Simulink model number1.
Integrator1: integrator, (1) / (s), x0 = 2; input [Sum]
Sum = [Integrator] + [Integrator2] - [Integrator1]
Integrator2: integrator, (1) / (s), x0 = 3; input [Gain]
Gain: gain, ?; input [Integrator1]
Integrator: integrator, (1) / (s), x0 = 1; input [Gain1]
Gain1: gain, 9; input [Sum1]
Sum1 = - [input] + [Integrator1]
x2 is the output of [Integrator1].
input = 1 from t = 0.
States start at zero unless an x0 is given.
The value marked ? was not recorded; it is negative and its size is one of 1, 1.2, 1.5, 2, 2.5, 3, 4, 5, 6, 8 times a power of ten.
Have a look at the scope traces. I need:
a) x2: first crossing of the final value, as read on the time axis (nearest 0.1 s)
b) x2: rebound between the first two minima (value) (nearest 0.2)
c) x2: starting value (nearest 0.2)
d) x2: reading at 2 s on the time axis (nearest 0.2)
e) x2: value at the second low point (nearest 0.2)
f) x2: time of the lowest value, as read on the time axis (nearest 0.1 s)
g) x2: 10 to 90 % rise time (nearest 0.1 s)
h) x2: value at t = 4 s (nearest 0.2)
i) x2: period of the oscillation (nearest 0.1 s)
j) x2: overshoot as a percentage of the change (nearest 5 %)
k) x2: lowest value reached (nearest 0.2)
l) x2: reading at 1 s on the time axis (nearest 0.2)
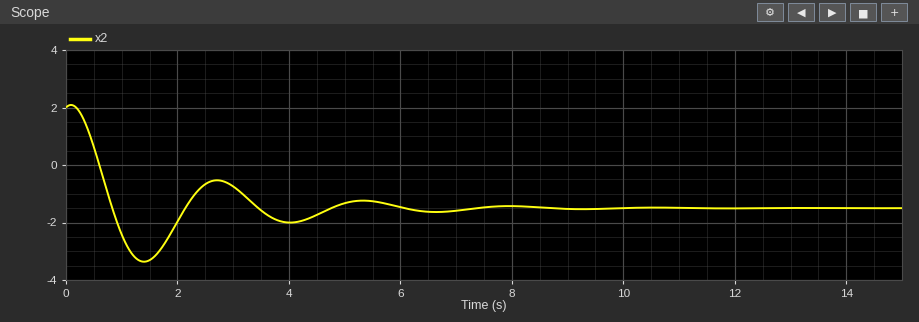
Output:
0.8 s
-0.6
2.0
-2.0
-2.0
1.4 s
0.5 s
-2.0
2.6 s
55 %
-3.4
-2.4
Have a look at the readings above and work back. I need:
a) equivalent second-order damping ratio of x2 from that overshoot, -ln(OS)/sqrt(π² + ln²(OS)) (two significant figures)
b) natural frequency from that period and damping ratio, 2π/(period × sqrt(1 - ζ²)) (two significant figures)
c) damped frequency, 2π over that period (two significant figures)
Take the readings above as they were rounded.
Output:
0.19
2.5 rad/s
2.4 rad/s
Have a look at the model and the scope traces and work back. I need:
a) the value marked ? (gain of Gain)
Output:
-15
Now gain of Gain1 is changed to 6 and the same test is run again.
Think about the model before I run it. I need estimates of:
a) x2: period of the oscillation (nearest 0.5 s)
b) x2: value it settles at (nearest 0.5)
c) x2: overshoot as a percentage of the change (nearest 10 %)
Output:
2.0 s
-0.5
60 %
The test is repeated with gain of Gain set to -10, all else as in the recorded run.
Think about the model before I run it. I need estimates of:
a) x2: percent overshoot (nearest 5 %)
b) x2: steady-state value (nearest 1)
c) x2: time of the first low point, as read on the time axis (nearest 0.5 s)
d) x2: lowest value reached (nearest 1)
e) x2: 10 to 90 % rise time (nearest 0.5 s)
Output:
15 %
-9
4.0 s
-11
1.5 s
